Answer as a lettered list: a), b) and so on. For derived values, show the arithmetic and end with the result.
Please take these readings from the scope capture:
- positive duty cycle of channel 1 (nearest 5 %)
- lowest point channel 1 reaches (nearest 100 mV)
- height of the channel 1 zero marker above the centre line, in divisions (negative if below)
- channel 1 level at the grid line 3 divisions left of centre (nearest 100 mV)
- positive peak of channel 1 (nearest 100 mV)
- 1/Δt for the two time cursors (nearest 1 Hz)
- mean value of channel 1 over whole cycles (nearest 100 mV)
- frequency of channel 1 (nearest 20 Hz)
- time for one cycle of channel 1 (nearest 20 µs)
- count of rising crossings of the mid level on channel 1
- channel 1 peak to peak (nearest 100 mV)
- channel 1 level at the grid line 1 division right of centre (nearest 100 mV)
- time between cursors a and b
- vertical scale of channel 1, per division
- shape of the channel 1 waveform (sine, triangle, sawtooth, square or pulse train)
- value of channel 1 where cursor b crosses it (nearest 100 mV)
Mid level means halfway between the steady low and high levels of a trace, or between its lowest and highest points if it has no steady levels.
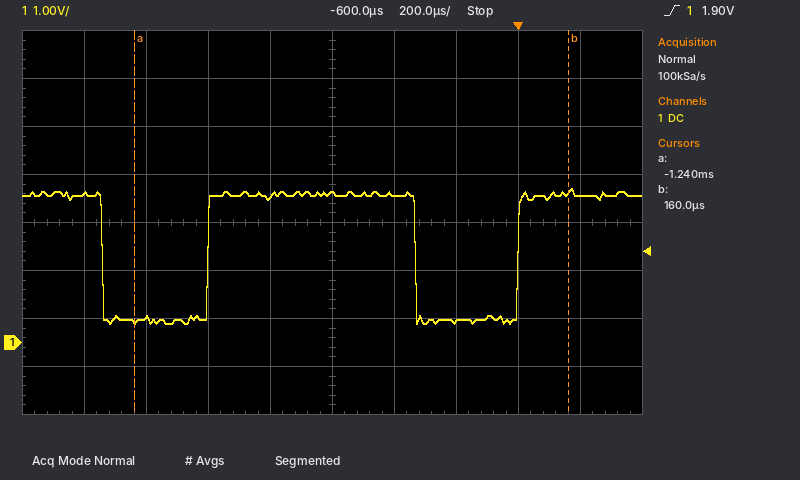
a) 65 %
b) 400 mV
c) -2.5 div
d) 500 mV
e) 3.2 V
f) 1 / 1.40 ms ≈ 714 Hz
g) 400 mV + 0.65 × (3.2 V − (400 mV)) ≈ 2.2 V
h) 1 / 1.00 ms ≈ 1.00 kHz
i) 1.00 ms
j) 2
k) 3.2 V − (400 mV) = 2.8 V
l) 3.1 V
m) 160 µs − (-1.24 ms) = 1.40 ms
n) 1 V
o) pulse train
p) 3.1 V
